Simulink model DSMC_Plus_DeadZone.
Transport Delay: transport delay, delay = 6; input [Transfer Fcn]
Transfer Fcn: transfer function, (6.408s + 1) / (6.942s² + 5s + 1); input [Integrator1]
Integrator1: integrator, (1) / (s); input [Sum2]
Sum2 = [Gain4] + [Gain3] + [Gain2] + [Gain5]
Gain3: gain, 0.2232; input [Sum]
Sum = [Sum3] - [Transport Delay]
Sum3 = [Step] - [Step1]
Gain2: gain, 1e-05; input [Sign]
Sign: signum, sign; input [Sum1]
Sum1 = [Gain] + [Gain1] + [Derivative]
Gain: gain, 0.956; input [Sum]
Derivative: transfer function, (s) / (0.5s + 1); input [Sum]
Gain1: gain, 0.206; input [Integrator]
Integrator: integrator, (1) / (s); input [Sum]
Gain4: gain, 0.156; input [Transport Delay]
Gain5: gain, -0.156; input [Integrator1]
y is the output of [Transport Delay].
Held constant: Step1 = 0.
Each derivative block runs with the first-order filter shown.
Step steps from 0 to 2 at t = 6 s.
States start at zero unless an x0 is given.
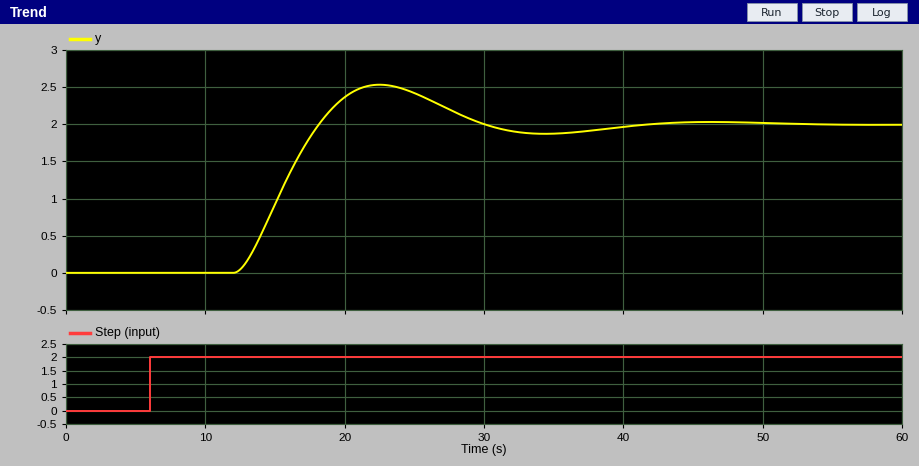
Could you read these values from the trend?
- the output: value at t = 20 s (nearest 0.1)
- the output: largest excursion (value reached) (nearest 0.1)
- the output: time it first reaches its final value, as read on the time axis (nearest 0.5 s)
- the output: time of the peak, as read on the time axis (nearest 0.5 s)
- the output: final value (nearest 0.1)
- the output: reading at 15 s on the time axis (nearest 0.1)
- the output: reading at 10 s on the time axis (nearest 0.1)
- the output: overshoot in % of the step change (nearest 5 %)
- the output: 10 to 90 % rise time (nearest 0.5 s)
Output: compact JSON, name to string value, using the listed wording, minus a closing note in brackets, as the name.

{"the output: value at t = 20 s": "2.4", "the output: largest excursion (value reached)": "2.5", "the output: time it first reaches its final value, as read on the time axis": "18.0 s", "the output: time of the peak, as read on the time axis": "22.5 s", "the output: final value": "2.0", "the output: reading at 15 s on the time axis": "0.9", "the output: reading at 10 s on the time axis": "0.0", "the output: overshoot in % of the step change": "25 %", "the output: 10 to 90 % rise time": "4.5 s"}
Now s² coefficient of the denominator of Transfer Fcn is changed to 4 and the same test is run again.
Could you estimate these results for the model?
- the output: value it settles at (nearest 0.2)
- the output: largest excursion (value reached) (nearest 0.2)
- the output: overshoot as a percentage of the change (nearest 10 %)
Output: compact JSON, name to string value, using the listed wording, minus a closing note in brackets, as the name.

{"the output: value it settles at": "2.0", "the output: largest excursion (value reached)": "2.4", "the output: overshoot as a percentage of the change": "20 %"}
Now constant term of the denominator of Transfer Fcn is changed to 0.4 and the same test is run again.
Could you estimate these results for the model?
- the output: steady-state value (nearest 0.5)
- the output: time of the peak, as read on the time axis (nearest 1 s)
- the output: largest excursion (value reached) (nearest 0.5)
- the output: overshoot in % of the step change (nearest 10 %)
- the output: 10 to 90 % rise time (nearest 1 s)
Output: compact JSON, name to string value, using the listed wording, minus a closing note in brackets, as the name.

{"the output: steady-state value": "3.5", "the output: time of the peak, as read on the time axis": "27 s", "the output: largest excursion (value reached)": "4.0", "the output: overshoot in % of the step change": "20 %", "the output: 10 to 90 % rise time": "6 s"}
